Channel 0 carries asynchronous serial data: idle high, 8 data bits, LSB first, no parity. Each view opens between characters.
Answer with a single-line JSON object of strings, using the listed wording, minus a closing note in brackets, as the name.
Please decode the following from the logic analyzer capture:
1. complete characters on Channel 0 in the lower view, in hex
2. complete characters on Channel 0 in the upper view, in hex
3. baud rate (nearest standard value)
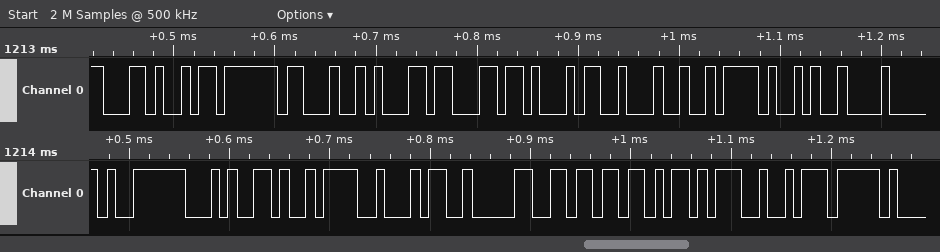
{"complete characters on Channel 0 in the lower view, in hex": "F9, 94, E9, A2, 82, B6, 6B, 27, F7", "complete characters on Channel 0 in the upper view, in hex": "2C, FB, 23, B1, 6C, 34, 24, 2F, 09", "baud rate": "115200 baud"}
